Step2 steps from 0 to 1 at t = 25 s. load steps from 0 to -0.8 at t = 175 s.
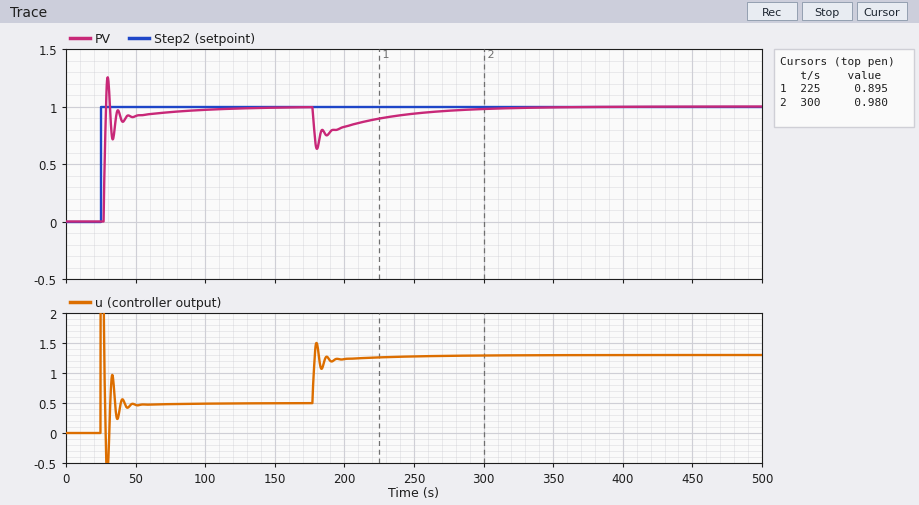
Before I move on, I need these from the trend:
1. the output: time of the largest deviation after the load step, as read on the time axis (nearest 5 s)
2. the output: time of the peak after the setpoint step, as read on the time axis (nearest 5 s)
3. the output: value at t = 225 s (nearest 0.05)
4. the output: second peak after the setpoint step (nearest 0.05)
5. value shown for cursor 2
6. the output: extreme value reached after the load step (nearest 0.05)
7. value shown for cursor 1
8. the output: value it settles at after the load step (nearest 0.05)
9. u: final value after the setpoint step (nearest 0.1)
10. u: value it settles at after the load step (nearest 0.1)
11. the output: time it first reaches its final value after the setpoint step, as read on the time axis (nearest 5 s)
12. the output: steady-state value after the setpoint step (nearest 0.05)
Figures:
180 s
30 s
0.90
0.95
0.980
0.65
0.895
1.00
0.5
1.3
30 s
1.00
